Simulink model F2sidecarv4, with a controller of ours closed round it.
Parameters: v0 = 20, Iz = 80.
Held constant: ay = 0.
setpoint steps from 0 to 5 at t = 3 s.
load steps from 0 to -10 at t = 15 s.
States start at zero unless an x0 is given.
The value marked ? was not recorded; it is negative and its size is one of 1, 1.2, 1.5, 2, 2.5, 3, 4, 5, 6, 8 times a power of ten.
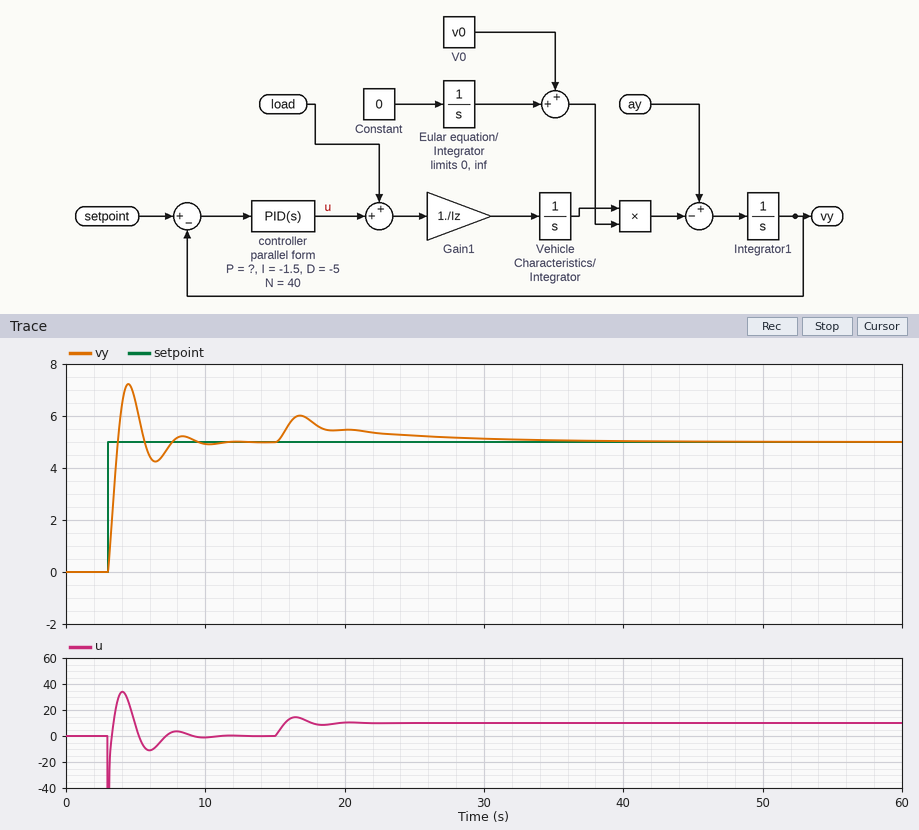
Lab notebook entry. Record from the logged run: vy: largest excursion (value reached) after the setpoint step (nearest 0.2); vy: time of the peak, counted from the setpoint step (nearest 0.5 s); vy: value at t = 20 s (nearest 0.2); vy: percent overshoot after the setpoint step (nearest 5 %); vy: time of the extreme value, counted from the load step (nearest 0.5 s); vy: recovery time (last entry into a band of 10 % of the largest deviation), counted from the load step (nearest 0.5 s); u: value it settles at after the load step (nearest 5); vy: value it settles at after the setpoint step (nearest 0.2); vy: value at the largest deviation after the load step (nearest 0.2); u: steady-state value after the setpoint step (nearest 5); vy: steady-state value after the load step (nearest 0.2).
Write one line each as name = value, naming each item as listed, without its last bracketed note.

vy: largest excursion (value reached) after the setpoint step = 7.2
vy: time of the peak, counted from the setpoint step = 1.5 s
vy: value at t = 20 s = 5.4
vy: percent overshoot after the setpoint step = 45 %
vy: time of the extreme value, counted from the load step = 2.0 s
vy: recovery time (last entry into a band of 10 % of the largest deviation), counted from the load step = 16.5 s
u: value it settles at after the load step = 10
vy: value it settles at after the setpoint step = 5.0
vy: value at the largest deviation after the load step = 6.0
u: steady-state value after the setpoint step = 0
vy: steady-state value after the load step = 5.0
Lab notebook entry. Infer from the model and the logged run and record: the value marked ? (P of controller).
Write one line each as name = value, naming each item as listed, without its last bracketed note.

the value marked ? = -12
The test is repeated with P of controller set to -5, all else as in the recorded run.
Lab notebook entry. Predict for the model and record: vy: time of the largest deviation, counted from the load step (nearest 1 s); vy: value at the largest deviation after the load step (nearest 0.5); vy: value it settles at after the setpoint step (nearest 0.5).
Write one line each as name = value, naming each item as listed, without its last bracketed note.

vy: time of the largest deviation, counted from the load step = 3 s
vy: value at the largest deviation after the load step = 7.0
vy: value it settles at after the setpoint step = 5.0
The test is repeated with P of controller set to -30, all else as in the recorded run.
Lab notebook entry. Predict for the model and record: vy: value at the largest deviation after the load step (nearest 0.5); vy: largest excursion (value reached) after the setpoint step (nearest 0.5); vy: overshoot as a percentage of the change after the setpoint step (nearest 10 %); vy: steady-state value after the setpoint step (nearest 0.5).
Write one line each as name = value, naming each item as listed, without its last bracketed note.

vy: value at the largest deviation after the load step = 5.5
vy: largest excursion (value reached) after the setpoint step = 8.0
vy: overshoot as a percentage of the change after the setpoint step = 60 %
vy: steady-state value after the setpoint step = 5.0
